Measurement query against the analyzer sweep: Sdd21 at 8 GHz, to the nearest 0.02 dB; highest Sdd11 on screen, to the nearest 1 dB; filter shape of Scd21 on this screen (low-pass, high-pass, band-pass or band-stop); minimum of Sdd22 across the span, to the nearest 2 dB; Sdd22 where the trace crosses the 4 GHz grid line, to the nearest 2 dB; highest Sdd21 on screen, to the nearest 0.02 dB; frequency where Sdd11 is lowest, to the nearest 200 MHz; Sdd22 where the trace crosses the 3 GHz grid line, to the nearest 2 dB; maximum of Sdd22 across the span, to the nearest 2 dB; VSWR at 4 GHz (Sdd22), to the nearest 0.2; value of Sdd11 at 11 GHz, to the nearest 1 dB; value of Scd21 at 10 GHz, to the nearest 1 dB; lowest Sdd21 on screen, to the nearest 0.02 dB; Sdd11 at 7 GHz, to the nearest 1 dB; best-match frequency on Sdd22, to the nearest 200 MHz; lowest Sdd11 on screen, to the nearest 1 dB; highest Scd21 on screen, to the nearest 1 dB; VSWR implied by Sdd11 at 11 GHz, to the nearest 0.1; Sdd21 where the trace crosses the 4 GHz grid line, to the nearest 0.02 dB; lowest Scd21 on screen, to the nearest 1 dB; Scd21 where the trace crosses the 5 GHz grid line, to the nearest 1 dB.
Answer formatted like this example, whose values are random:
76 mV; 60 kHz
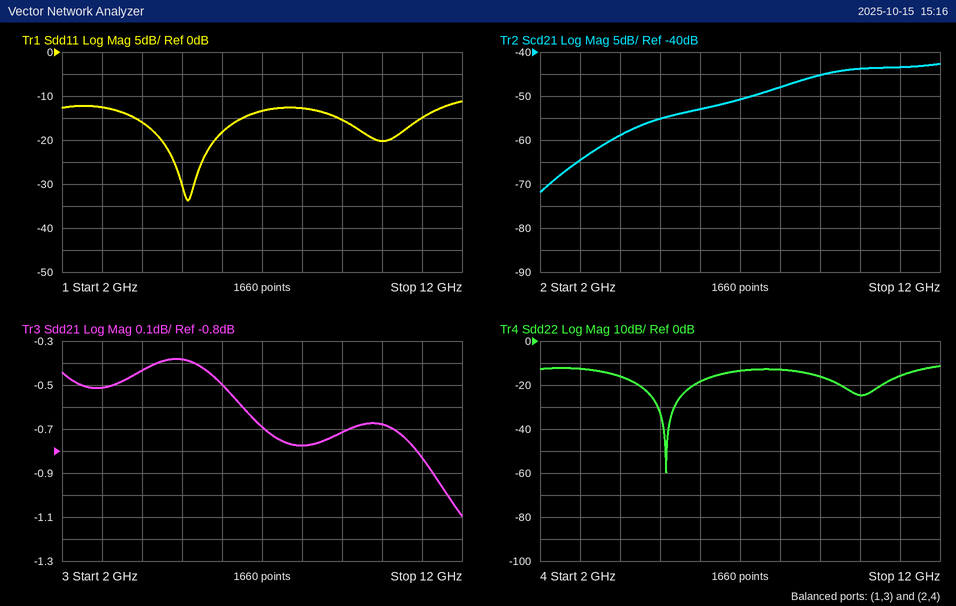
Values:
-0.78 dB; -11 dB; high-pass; -60 dB; -16 dB; -0.38 dB; 5.2 GHz; -12 dB; -12 dB; 1.4; -15 dB; -44 dB; -1.10 dB; -13 dB; 5.2 GHz; -34 dB; -43 dB; 1.4; -0.44 dB; -72 dB; -55 dB
